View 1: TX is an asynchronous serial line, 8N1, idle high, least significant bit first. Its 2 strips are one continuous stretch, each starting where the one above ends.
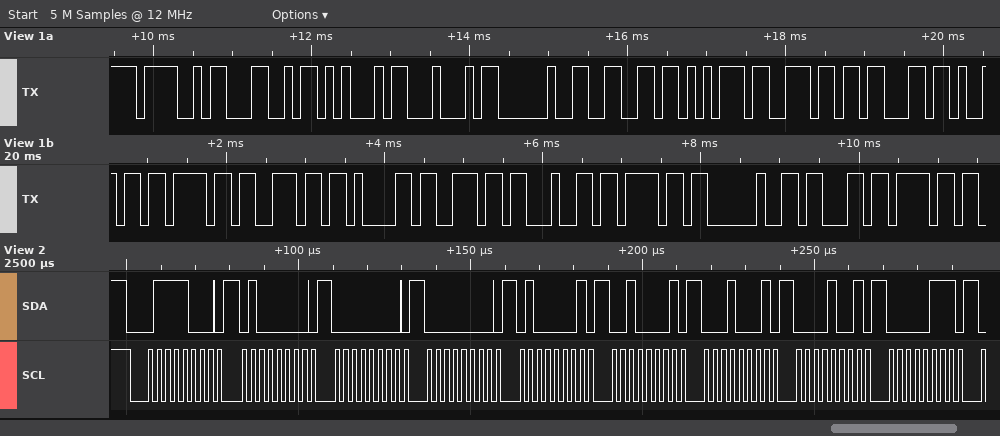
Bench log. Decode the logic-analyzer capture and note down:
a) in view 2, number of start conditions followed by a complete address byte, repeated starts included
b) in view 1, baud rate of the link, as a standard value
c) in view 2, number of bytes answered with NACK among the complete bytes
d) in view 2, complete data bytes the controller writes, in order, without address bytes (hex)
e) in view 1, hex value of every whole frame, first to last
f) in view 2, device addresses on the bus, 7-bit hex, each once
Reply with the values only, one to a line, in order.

1
9600 baud
0
40 00 00 41 21 11 09 07
4F 4C 45 44 20 66 75 6E 63 69 6F 6E 61 6E 64 6F 20 63 6F
0x3C
